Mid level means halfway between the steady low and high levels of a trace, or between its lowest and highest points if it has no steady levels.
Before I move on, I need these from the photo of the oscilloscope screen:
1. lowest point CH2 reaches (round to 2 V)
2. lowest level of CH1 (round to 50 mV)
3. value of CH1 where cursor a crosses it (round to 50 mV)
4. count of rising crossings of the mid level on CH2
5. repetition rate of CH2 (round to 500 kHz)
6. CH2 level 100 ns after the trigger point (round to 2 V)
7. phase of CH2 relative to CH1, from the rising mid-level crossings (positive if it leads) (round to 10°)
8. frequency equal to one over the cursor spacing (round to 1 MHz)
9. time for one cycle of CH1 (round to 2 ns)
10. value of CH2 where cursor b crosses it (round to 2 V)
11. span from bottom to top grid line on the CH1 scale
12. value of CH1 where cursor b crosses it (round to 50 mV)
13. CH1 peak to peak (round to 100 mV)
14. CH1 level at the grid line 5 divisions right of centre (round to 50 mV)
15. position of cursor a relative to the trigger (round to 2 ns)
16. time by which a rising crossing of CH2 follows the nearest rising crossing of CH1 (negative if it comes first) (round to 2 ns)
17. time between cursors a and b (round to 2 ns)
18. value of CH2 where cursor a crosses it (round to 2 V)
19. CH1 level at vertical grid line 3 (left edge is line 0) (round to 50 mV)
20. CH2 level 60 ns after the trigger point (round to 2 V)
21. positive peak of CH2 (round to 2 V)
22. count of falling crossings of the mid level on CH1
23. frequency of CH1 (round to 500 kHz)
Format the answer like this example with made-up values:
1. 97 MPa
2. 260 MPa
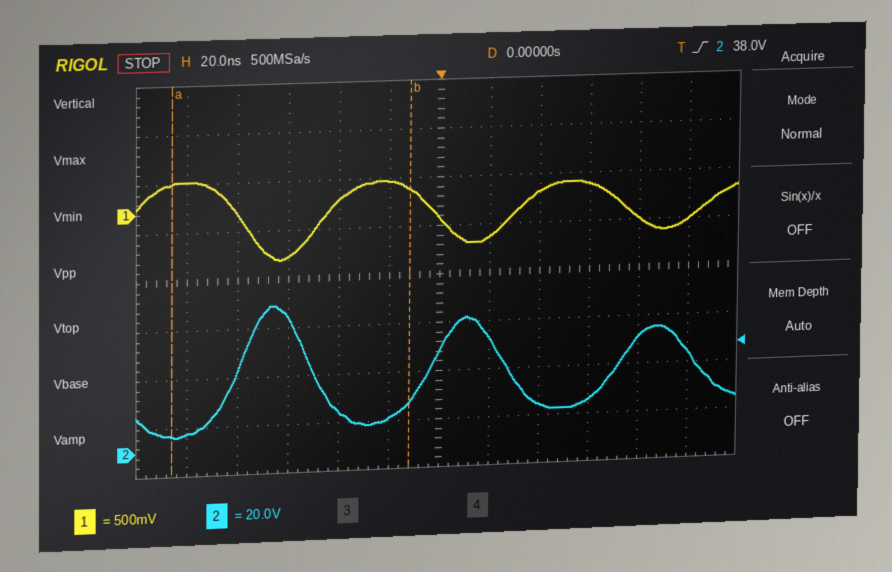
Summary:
1. 6 V
2. -500 mV
3. 300 mV
4. 3
5. 13.0 MHz
6. 34 V
7. +150°
8. 11 MHz
9. 76 ns
10. 18 V
11. 4 V
12. 200 mV
13. 800 mV
14. -200 mV
15. -106 ns
16. -32 ns
17. 94 ns
18. 6 V
19. -450 mV
20. 16 V
21. 60 V
22. 3
23. 13.0 MHz
